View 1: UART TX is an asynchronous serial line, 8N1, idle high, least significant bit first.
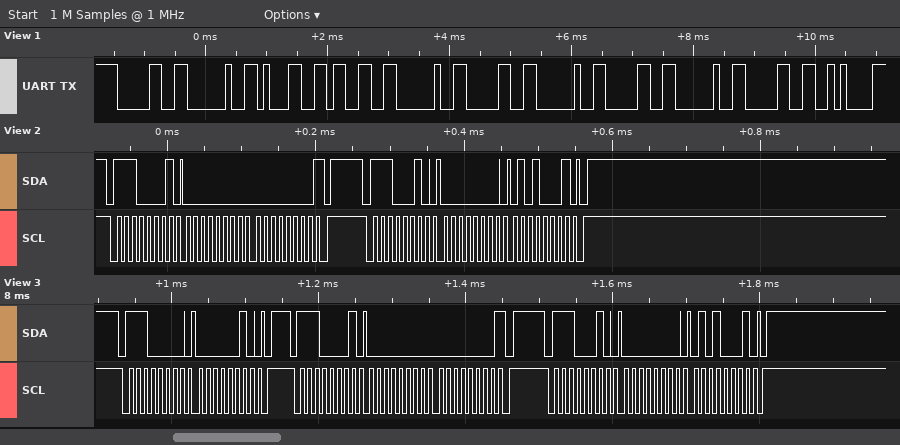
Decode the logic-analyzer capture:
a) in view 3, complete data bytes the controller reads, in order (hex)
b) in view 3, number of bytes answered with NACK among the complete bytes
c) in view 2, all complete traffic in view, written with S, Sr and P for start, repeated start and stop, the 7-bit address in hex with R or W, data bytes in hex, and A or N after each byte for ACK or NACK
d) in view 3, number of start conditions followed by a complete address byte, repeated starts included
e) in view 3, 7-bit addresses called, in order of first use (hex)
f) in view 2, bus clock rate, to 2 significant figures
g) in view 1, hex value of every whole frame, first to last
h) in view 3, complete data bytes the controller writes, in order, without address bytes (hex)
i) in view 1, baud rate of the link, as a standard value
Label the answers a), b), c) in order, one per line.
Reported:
a) 00 00
b) 1
c) S 70R A 00 A 00 N P S 71W A 00 A 51 A P
d) 3
e) 0x70 0x71
f) 100 kHz
g) 0x30 0x20 0x31 0x33 0x20 0x30 0x20 0x30 0x20 0x30 0x0A
h) 02 00 51
i) 9600 baud
